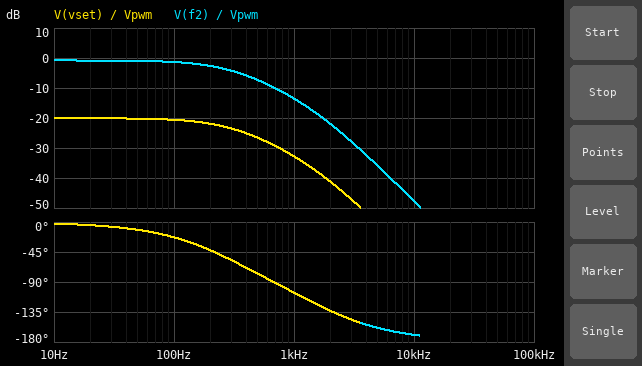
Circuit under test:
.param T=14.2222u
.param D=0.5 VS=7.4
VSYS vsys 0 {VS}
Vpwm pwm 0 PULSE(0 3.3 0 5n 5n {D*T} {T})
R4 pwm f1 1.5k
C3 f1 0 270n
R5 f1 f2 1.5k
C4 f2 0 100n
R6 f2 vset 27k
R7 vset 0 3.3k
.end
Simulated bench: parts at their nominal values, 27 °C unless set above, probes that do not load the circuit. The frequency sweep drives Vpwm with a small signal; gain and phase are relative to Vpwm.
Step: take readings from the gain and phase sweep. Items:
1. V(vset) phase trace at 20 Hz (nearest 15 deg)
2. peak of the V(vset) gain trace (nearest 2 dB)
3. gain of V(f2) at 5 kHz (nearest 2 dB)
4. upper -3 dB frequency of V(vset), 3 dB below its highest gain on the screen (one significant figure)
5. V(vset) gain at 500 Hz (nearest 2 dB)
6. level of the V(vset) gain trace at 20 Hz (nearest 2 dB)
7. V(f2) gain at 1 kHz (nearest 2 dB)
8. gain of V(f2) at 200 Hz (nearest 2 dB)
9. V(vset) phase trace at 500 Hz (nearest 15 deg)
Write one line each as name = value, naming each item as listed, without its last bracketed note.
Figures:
V(vset) phase trace at 20 Hz = 0 deg
peak of the V(vset) gain trace = -20 dB
gain of V(f2) at 5 kHz = -36 dB
upper -3 dB frequency of V(vset), 3 dB below its highest gain on the screen = 300 Hz
V(vset) gain at 500 Hz = -26 dB
level of the V(vset) gain trace at 20 Hz = -20 dB
V(f2) gain at 1 kHz = -14 dB
gain of V(f2) at 200 Hz = -2 dB
V(vset) phase trace at 500 Hz = -75 deg
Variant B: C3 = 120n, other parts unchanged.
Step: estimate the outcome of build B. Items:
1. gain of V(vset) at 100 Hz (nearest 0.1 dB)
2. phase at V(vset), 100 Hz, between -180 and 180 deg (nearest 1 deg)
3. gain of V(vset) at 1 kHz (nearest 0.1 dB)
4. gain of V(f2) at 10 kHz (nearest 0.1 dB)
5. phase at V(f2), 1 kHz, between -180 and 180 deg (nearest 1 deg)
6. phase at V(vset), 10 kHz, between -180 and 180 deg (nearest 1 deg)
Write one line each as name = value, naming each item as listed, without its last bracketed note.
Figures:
gain of V(vset) at 100 Hz = -20.3 dB
phase at V(vset), 100 Hz, between -180 and 180 deg = -16 deg
gain of V(vset) at 1 kHz = -29.0 dB
gain of V(f2) at 10 kHz = -40.8 dB
phase at V(f2), 1 kHz, between -180 and 180 deg = -89 deg
phase at V(vset), 10 kHz, between -180 and 180 deg = -164 deg
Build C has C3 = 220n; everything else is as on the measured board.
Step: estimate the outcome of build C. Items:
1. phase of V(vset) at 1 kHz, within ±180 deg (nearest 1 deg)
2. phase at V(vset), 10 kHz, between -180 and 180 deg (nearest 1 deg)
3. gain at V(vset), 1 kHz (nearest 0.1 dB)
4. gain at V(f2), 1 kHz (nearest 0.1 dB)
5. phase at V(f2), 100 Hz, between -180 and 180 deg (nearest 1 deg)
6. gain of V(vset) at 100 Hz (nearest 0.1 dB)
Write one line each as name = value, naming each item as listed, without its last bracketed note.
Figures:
phase of V(vset) at 1 kHz, within ±180 deg = -102 deg
phase at V(vset), 10 kHz, between -180 and 180 deg = -168 deg
gain at V(vset), 1 kHz = -31.6 dB
gain at V(f2), 1 kHz = -12.4 dB
phase at V(f2), 100 Hz, between -180 and 180 deg = -21 deg
gain of V(vset) at 100 Hz = -20.5 dB
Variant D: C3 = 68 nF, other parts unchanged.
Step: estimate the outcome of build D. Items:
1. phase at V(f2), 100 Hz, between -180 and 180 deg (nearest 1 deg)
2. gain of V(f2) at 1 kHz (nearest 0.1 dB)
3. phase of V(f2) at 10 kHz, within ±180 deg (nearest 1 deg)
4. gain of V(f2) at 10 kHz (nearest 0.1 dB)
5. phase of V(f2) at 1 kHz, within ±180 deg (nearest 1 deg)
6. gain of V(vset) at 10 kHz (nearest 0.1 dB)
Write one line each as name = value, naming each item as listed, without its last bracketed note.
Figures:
phase at V(f2), 100 Hz, between -180 and 180 deg = -13 deg
gain of V(f2) at 1 kHz = -8.3 dB
phase of V(f2) at 10 kHz, within ±180 deg = -157 deg
gain of V(f2) at 10 kHz = -36.2 dB
phase of V(f2) at 1 kHz, within ±180 deg = -79 deg
gain of V(vset) at 10 kHz = -55.5 dB
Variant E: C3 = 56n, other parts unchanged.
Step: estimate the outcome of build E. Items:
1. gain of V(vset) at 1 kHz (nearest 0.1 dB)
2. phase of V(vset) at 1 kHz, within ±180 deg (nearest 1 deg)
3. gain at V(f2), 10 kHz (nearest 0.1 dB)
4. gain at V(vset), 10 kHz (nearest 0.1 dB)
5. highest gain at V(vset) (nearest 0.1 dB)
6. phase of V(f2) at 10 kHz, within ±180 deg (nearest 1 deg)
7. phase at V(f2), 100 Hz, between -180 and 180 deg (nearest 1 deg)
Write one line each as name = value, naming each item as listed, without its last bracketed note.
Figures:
gain of V(vset) at 1 kHz = -27.3 dB
phase of V(vset) at 1 kHz, within ±180 deg = -76 deg
gain at V(f2), 10 kHz = -34.7 dB
gain at V(vset), 10 kHz = -54.0 dB
highest gain at V(vset) = -20.1 dB
phase of V(f2) at 10 kHz, within ±180 deg = -153 deg
phase at V(f2), 100 Hz, between -180 and 180 deg = -13 deg
